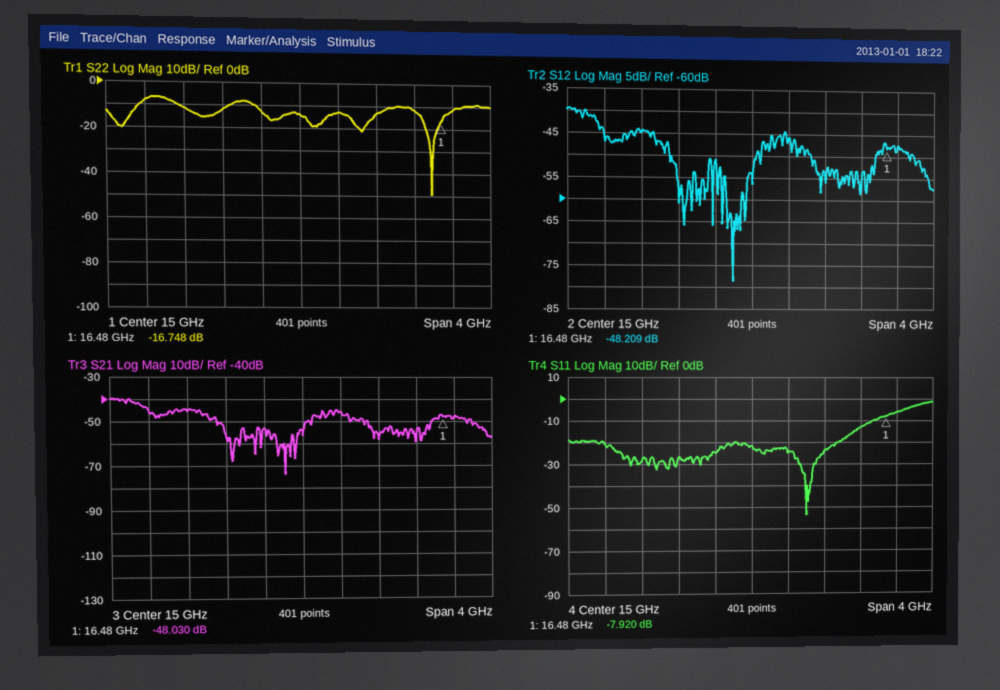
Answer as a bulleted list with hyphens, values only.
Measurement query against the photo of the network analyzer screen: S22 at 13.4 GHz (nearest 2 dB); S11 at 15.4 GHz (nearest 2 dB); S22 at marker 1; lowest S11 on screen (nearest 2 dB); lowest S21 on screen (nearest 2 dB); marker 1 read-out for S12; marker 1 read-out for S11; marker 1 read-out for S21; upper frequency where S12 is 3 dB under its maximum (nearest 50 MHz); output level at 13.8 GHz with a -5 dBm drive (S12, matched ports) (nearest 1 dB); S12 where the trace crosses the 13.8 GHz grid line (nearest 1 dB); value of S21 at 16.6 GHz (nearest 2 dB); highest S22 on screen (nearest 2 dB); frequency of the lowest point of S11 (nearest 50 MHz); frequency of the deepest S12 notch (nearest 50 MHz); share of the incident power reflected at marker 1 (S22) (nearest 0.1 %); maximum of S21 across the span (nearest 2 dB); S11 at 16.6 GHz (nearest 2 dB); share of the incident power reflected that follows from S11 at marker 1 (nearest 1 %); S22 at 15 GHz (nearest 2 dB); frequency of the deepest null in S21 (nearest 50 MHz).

- -8 dB
- -24 dB
- -16.748 dB
- -54 dB
- -74 dB
- -48.209 dB
- -7.920 dB
- -48.030 dB
- 13.30 GHz
- -50 dBm
- -45 dB
- -48 dB
- -6 dB
- 15.60 GHz
- 14.80 GHz
- 2.1 %
- -40 dB
- -6 dB
- 16 %
- -14 dB
- 14.80 GHz
